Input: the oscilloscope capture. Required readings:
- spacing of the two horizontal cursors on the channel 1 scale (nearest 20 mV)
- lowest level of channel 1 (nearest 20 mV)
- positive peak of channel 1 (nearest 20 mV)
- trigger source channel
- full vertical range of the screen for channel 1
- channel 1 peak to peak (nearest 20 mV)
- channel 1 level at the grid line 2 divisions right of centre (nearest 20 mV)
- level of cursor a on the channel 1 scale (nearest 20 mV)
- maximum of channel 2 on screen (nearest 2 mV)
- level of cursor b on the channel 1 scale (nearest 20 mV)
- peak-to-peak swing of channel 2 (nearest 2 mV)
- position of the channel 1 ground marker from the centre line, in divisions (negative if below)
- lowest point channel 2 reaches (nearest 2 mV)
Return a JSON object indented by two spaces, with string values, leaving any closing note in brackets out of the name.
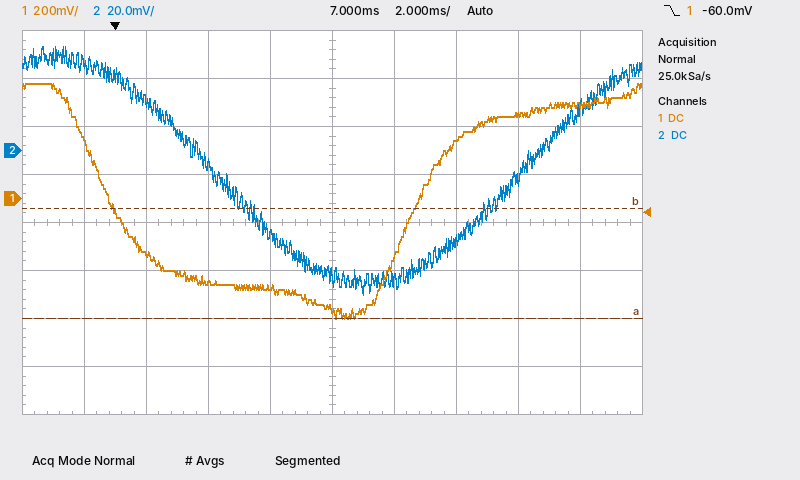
{
  "spacing of the two horizontal cursors on the channel 1 scale": "460 mV",
  "lowest level of channel 1": "-500 mV",
  "positive peak of channel 1": "480 mV",
  "trigger source channel": "channel 1",
  "full vertical range of the screen for channel 1": "1.6 V",
  "channel 1 peak to peak": "980 mV",
  "channel 1 level at the grid line 2 divisions right of centre": "240 mV",
  "level of cursor a on the channel 1 scale": "-500 mV",
  "maximum of channel 2 on screen": "44 mV",
  "level of cursor b on the channel 1 scale": "-40 mV",
  "peak-to-peak swing of channel 2": "104 mV",
  "position of the channel 1 ground marker from the centre line, in divisions": "+0.5 div",
  "lowest point channel 2 reaches": "-60 mV"
}
